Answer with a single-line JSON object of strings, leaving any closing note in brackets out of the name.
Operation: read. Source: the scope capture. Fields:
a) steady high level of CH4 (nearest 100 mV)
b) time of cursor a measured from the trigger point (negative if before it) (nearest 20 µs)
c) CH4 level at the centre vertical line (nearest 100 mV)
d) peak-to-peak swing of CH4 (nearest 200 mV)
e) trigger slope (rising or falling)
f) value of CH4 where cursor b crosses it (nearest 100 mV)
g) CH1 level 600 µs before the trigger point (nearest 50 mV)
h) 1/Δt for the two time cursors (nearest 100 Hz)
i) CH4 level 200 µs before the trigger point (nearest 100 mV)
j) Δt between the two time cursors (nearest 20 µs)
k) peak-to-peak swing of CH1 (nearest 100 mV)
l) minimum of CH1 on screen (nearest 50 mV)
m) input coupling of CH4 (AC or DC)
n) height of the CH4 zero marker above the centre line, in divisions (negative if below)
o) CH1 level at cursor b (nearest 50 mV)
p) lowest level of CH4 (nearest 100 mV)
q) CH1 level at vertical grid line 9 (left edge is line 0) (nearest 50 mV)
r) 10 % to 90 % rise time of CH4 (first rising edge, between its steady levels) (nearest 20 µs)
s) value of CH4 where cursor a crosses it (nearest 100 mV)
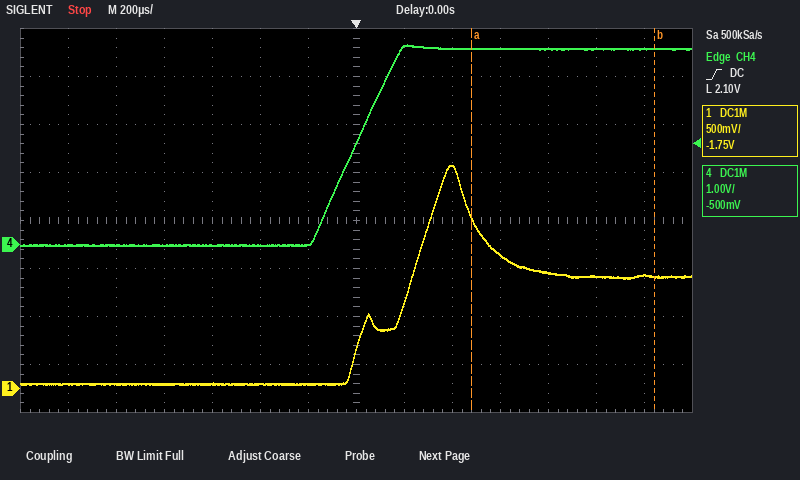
{"steady high level of CH4": "4.1 V", "time of cursor a measured from the trigger point (negative if before it)": "+480 µs", "CH4 level at the centre vertical line": "2.1 V", "peak-to-peak swing of CH4": "4.2 V", "trigger slope": "rising", "value of CH4 where cursor b crosses it": "4.1 V", "CH1 level 600 µs before the trigger point": "50 mV", "1/Δt for the two time cursors": "1.3 kHz", "CH4 level 200 µs before the trigger point": "0.0 V", "Δt between the two time cursors": "760 µs", "peak-to-peak swing of CH1": "2.30 V", "minimum of CH1 on screen": "50 mV", "input coupling of CH4": "DC", "height of the CH4 zero marker above the centre line, in divisions": "-0.5 div", "CH1 level at cursor b": "1.15 V", "lowest level of CH4": "0.0 V", "CH1 level at vertical grid line 9 (left edge is line 0)": "2.30 V", "10 % to 90 % rise time of CH4 (first rising edge, between its steady levels)": "300 µs", "value of CH4 where cursor a crosses it": "4.1 V"}
